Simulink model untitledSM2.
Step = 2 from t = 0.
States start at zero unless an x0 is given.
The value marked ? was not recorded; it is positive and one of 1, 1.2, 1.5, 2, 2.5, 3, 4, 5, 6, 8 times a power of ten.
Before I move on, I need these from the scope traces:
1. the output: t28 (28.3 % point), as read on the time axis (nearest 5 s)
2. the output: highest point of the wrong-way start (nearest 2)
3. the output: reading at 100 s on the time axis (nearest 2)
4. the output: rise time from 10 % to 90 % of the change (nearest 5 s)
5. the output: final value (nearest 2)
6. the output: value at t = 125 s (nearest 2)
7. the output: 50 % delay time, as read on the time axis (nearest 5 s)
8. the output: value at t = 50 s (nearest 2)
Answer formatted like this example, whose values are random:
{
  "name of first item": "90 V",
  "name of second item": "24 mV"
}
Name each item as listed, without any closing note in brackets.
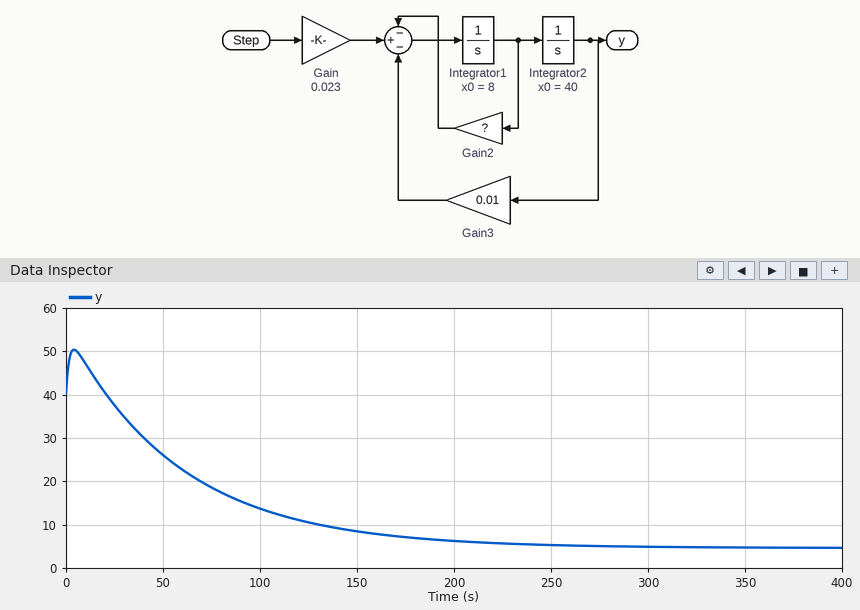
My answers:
{
  "the output: t28 (28.3 % point), as read on the time axis": "40 s",
  "the output: highest point of the wrong-way start": "50",
  "the output: reading at 100 s on the time axis": "14",
  "the output: rise time from 10 % to 90 % of the change": "130 s",
  "the output: final value": "4",
  "the output: value at t = 125 s": "10",
  "the output: 50 % delay time, as read on the time axis": "60 s",
  "the output: value at t = 50 s": "26"
}
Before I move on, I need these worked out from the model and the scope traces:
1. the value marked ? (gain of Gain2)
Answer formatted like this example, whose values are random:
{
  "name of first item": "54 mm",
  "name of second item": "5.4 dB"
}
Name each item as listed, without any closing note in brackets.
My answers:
{
  "the value marked ?": "0.6"
}
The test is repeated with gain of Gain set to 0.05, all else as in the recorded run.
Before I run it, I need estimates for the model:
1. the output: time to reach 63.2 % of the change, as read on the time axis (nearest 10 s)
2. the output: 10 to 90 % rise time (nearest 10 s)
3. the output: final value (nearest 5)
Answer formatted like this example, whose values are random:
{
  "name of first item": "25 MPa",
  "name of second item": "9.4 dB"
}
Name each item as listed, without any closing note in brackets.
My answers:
{
  "the output: time to reach 63.2 % of the change, as read on the time axis": "80 s",
  "the output: 10 to 90 % rise time": "130 s",
  "the output: final value": "10"
}
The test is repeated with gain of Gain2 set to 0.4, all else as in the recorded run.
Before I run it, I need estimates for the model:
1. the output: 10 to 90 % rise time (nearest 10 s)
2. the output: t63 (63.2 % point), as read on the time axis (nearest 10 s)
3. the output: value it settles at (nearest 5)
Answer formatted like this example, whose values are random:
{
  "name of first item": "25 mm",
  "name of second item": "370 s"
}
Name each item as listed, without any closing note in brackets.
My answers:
{
  "the output: 10 to 90 % rise time": "80 s",
  "the output: t63 (63.2 % point), as read on the time axis": "60 s",
  "the output: value it settles at": "5"
}
